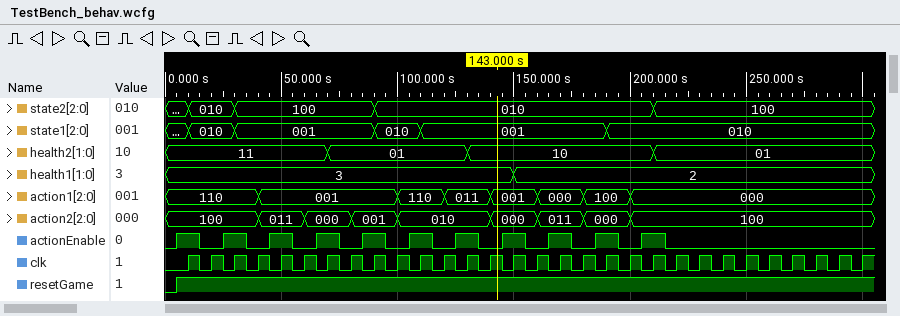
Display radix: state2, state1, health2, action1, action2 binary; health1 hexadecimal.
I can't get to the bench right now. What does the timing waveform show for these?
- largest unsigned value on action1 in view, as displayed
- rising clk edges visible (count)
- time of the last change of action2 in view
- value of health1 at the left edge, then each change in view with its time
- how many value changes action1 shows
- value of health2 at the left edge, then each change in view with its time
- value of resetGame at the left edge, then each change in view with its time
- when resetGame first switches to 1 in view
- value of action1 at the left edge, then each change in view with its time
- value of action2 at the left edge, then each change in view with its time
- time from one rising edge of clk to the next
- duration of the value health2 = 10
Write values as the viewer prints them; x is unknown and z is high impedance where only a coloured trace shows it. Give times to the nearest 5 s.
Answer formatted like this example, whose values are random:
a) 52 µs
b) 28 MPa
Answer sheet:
a) 110
b) 30
c) 200 s
d) 3, 2 at 150 s
e) 7
f) 11, 01 at 70 s, 10 at 130 s, 01 at 210 s
g) 0, 1 at 5 s
h) 5 s
i) 110, 001 at 40 s, 110 at 100 s, 011 at 120 s, 001 at 140 s, 000 at 160 s, 100 at 180 s, 000 at 200 s
j) 100, 011 at 40 s, 000 at 60 s, 001 at 80 s, 010 at 100 s, 000 at 140 s, 011 at 160 s, 000 at 180 s, 100 at 200 s
k) 10 s
l) 80 s
